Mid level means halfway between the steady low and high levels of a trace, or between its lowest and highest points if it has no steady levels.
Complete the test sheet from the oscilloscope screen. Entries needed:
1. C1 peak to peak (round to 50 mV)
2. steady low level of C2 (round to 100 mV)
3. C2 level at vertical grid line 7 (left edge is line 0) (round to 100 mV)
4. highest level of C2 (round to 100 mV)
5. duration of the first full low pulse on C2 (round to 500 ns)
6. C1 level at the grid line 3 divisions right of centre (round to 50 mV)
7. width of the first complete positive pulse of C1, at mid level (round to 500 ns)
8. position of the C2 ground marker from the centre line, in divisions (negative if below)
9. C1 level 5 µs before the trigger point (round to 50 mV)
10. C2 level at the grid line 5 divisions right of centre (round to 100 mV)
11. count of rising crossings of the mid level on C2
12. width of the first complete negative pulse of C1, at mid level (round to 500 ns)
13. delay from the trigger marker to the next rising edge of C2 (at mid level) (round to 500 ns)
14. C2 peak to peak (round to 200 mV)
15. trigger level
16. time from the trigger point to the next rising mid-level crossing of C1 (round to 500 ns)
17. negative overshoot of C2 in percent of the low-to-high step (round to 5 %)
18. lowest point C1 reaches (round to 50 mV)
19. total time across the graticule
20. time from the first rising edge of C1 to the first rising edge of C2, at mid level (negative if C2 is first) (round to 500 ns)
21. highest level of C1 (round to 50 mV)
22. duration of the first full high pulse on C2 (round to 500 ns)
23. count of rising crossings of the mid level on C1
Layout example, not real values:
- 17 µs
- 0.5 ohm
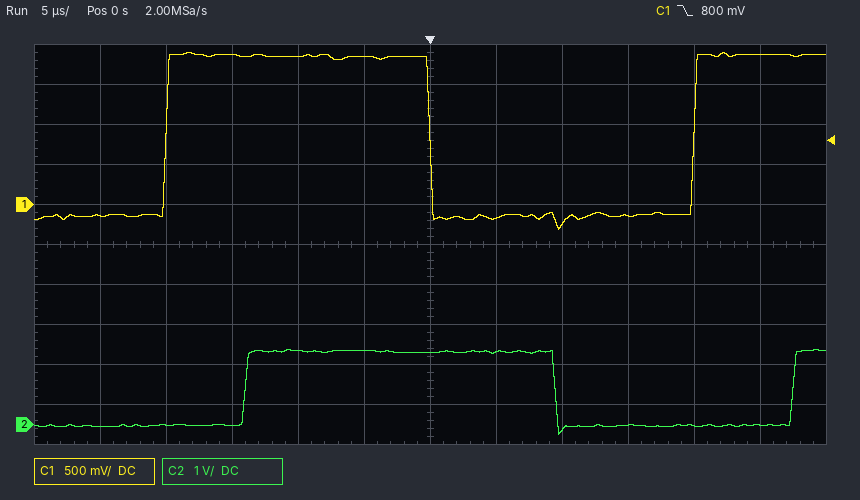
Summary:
- 2.20 V
- 0.0 V
- 1.8 V
- 1.9 V
- 18.0 µs
- -150 mV
- 20.0 µs
- -4.5 div
- 1.85 V
- 0.0 V
- 2
- 20.0 µs
- 27.5 µs
- 2.2 V
- 800 mV
- 20.0 µs
- 10 %
- -300 mV
- 60 µs
- +6.0 µs
- 1.90 V
- 23.5 µs
- 2
